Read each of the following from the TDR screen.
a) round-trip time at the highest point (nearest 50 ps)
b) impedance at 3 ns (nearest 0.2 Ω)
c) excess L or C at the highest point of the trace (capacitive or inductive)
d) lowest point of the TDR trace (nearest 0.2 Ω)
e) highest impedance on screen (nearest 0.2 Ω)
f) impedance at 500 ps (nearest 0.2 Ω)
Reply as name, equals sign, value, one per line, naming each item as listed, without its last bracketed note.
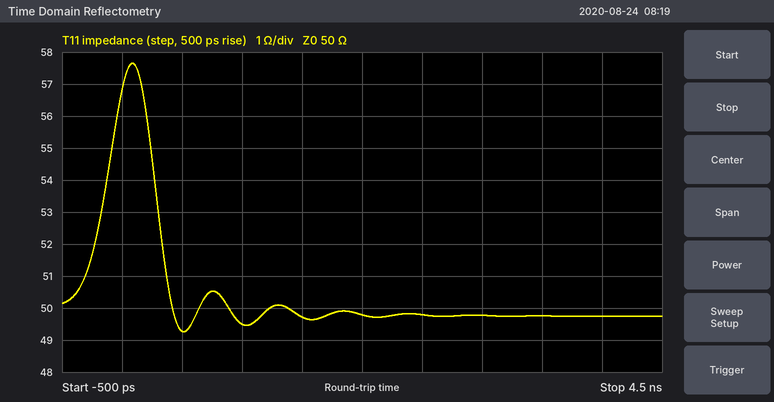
round-trip time at the highest point = 100 ps
impedance at 3 ns = 49.8 Ω
excess L or C at the highest point of the trace = inductive
lowest point of the TDR trace = 49.2 Ω
highest impedance on screen = 57.6 Ω
impedance at 500 ps = 49.2 Ω
